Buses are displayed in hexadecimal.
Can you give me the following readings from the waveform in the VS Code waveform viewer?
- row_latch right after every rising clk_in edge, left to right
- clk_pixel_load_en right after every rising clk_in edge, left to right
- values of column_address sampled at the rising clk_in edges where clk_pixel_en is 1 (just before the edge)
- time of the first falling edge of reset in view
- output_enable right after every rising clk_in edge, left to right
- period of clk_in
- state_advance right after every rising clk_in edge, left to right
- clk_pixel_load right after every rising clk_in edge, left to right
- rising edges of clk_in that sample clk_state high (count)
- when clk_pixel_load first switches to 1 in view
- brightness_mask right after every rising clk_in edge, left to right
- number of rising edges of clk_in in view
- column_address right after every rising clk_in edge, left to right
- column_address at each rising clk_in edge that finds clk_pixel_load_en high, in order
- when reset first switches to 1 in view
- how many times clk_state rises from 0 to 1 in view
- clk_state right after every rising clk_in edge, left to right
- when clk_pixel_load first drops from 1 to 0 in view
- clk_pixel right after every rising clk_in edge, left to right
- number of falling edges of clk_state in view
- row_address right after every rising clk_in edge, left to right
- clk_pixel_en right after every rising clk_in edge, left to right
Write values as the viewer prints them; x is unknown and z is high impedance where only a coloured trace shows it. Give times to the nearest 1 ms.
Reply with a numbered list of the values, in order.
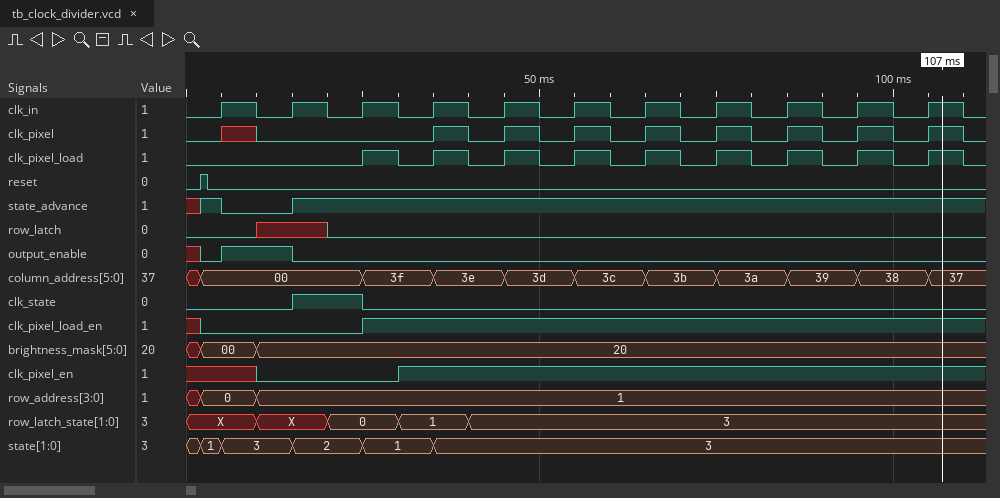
1. 0 x 0 0 0 0 0 0 0 0 0
2. 0 0 1 1 1 1 1 1 1 1 1
3. 3f, 3e, 3d, 3c, 3b, 3a, 39, 38
4. 3 ms
5. 1 0 0 0 0 0 0 0 0 0 0
6. 10 ms
7. 0 1 1 1 1 1 1 1 1 1 1
8. 0 0 1 1 1 1 1 1 1 1 1
9. 1
10. 25 ms
11. 00, 20, 20, 20, 20, 20, 20, 20, 20, 20, 20
12. 11
13. 00, 00, 3f, 3e, 3d, 3c, 3b, 3a, 39, 38, 37
14. 3f, 3e, 3d, 3c, 3b, 3a, 39, 38
15. 2 ms
16. 1
17. 0 1 0 0 0 0 0 0 0 0 0
18. 30 ms
19. x 0 0 1 1 1 1 1 1 1 1
20. 1
21. 0, 1, 1, 1, 1, 1, 1, 1, 1, 1, 1
22. x 0 0 1 1 1 1 1 1 1 1
